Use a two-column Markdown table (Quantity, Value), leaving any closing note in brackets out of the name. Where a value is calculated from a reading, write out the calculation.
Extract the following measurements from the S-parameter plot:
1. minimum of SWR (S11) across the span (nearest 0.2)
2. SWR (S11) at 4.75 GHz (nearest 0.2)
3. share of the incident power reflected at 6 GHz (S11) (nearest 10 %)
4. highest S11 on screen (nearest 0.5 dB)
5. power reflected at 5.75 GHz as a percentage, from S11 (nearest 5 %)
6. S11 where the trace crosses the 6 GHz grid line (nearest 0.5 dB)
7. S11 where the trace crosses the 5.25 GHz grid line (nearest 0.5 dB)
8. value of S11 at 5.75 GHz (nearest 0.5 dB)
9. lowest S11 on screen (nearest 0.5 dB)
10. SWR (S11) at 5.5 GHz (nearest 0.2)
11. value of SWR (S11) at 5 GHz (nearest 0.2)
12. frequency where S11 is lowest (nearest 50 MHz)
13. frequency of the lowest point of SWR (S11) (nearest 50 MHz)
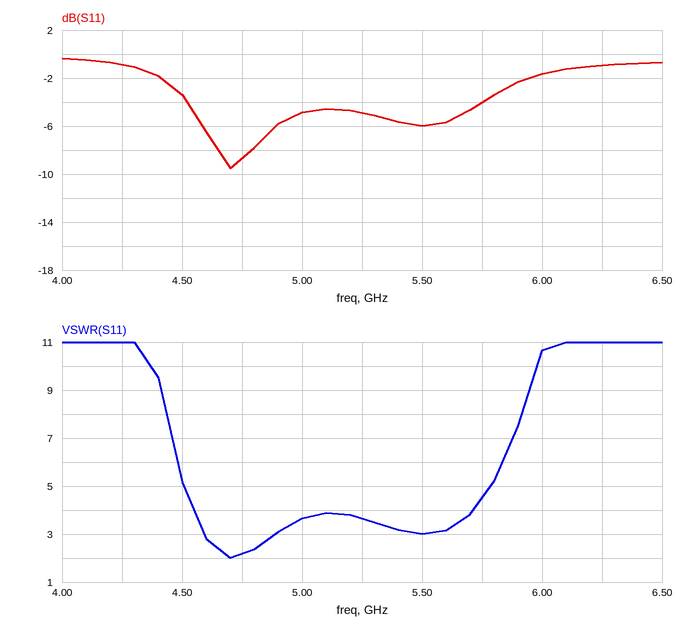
| Quantity | Value |
|---|---|
| minimum of SWR (S11) across the span | 2.0 |
| SWR (S11) at 4.75 GHz | 2.2 |
| share of the incident power reflected at 6 GHz (S11) | 10^(-1.5/10) ≈ 70.8 %, so 70 % to the nearest 10 % |
| highest S11 on screen | -0.5 dB |
| power reflected at 5.75 GHz as a percentage, from S11 | 10^(-4/10) ≈ 40 % |
| S11 where the trace crosses the 6 GHz grid line | -1.5 dB |
| S11 where the trace crosses the 5.25 GHz grid line | -5.0 dB |
| value of S11 at 5.75 GHz | -4.0 dB |
| lowest S11 on screen | -9.5 dB |
| SWR (S11) at 5.5 GHz | 3.0 |
| value of SWR (S11) at 5 GHz | 3.6 |
| frequency where S11 is lowest | 4.70 GHz |
| frequency of the lowest point of SWR (S11) | 4.70 GHz |
